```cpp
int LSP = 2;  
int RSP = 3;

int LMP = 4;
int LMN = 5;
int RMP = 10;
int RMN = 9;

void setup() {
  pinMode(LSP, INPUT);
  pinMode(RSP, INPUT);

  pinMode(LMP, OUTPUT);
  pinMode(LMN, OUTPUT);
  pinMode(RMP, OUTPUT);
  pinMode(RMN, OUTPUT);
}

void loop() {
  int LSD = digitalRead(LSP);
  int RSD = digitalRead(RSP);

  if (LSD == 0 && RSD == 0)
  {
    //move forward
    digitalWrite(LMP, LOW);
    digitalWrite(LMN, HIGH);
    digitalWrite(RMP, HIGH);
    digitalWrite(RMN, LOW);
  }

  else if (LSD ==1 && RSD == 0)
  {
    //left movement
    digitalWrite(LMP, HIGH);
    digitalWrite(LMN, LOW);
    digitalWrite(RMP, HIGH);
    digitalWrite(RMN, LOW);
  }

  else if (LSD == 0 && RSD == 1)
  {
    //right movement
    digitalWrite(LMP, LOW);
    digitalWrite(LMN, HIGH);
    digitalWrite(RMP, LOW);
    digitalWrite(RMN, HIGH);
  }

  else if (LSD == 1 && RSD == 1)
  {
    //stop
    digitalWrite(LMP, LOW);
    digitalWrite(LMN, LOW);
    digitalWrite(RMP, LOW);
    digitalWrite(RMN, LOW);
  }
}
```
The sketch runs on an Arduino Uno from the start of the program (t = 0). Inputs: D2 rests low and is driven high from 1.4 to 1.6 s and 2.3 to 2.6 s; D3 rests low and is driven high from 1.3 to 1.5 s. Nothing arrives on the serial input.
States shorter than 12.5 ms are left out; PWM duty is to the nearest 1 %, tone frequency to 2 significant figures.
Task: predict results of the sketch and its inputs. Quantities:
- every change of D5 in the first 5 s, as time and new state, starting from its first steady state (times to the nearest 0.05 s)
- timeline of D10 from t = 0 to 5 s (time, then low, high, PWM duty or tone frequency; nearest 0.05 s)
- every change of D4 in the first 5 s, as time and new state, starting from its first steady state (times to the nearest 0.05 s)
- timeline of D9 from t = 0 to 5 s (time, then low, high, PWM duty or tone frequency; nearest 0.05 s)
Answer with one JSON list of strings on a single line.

["0 s high; 1.4 s low; 1.6 s high; 2.3 s low; 2.6 s high", "0 s high; 1.3 s low; 1.5 s high", "0 s low; 1.5 s high; 1.6 s low; 2.3 s high; 2.6 s low", "0 s low; 1.3 s high; 1.4 s low"]
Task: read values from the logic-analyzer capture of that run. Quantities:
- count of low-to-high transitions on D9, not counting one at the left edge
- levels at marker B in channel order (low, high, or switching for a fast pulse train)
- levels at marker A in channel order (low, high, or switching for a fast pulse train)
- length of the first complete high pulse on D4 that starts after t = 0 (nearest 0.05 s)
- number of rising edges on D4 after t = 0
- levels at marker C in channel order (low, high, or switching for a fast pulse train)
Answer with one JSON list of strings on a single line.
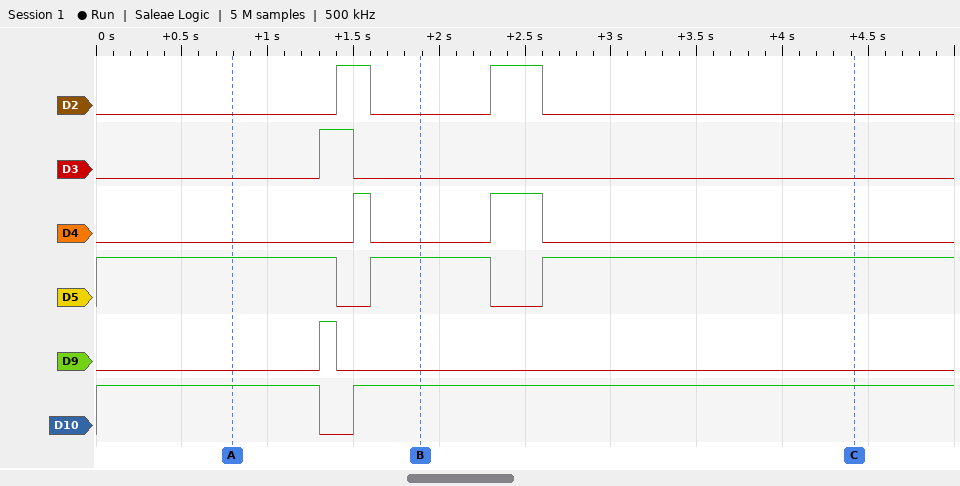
["1", "D2 low, D3 low, D4 low, D5 high, D9 low, D10 high", "D2 low, D3 low, D4 low, D5 high, D9 low, D10 high", "0.10 s", "2", "D2 low, D3 low, D4 low, D5 high, D9 low, D10 high"]
